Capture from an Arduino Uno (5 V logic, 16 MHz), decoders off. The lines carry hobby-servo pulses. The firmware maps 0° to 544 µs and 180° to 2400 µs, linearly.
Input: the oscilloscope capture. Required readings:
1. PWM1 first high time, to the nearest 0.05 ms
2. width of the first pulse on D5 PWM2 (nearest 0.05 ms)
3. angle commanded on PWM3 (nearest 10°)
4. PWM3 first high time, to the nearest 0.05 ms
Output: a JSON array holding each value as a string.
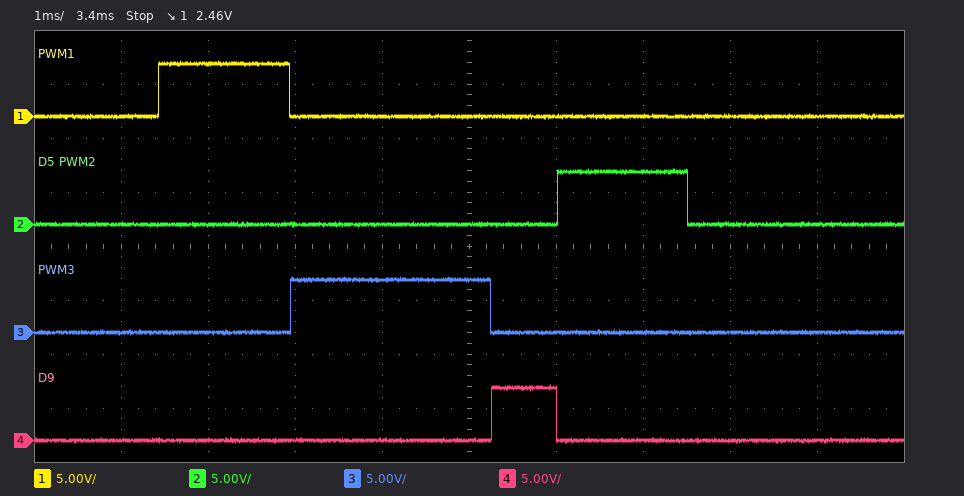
["1.50 ms", "1.50 ms", "170°", "2.30 ms"]
